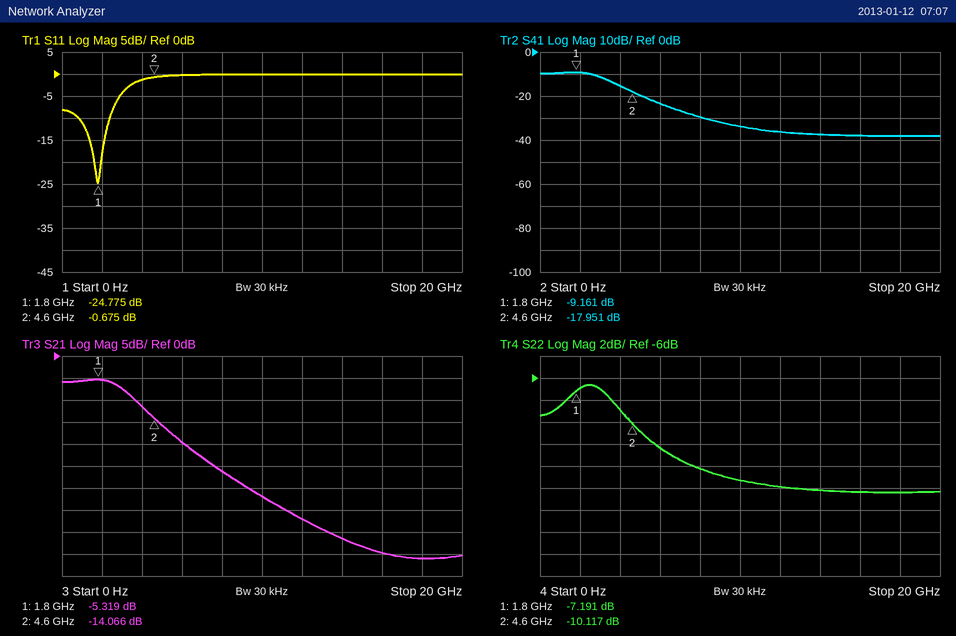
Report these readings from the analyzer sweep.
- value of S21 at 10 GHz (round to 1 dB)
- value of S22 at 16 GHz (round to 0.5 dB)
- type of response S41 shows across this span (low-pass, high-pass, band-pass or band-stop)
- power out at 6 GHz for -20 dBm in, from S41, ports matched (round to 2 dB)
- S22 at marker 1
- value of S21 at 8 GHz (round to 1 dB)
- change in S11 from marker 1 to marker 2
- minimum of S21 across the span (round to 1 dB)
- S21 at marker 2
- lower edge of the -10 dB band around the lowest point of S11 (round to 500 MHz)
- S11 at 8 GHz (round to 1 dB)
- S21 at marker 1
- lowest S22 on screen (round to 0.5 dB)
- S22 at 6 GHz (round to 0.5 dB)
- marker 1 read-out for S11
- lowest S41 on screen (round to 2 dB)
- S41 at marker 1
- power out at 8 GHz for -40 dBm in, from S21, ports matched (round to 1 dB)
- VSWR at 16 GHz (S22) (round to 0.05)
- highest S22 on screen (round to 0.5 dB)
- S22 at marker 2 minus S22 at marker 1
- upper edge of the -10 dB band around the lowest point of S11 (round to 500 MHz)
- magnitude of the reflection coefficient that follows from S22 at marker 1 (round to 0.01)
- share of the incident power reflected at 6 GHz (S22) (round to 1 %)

-32 dB
-16.5 dB
low-pass
-44 dBm
-7.191 dB
-26 dB
24.100 dB
-46 dB
-14.066 dB
1.0 GHz
0 dB
-5.319 dB
-16.5 dB
-12.5 dB
-24.775 dB
-38 dB
-9.161 dB
-66 dBm
1.35
-6.5 dB
-2.926 dB
2.5 GHz
0.44
6 %
